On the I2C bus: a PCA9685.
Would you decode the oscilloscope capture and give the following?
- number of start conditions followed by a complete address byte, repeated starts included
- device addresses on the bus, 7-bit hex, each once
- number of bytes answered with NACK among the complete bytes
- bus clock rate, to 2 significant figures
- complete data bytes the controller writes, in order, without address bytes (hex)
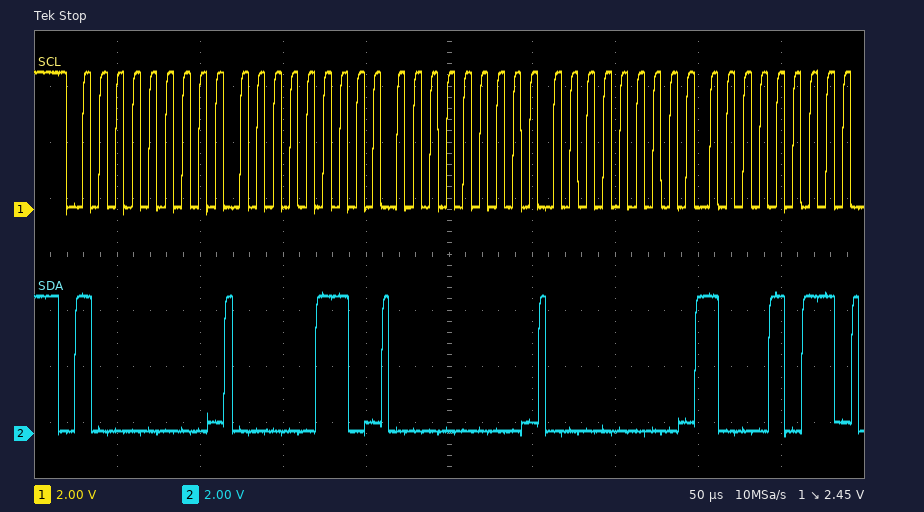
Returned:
1
0x40
0
100 kHz
06 00 00 8B
